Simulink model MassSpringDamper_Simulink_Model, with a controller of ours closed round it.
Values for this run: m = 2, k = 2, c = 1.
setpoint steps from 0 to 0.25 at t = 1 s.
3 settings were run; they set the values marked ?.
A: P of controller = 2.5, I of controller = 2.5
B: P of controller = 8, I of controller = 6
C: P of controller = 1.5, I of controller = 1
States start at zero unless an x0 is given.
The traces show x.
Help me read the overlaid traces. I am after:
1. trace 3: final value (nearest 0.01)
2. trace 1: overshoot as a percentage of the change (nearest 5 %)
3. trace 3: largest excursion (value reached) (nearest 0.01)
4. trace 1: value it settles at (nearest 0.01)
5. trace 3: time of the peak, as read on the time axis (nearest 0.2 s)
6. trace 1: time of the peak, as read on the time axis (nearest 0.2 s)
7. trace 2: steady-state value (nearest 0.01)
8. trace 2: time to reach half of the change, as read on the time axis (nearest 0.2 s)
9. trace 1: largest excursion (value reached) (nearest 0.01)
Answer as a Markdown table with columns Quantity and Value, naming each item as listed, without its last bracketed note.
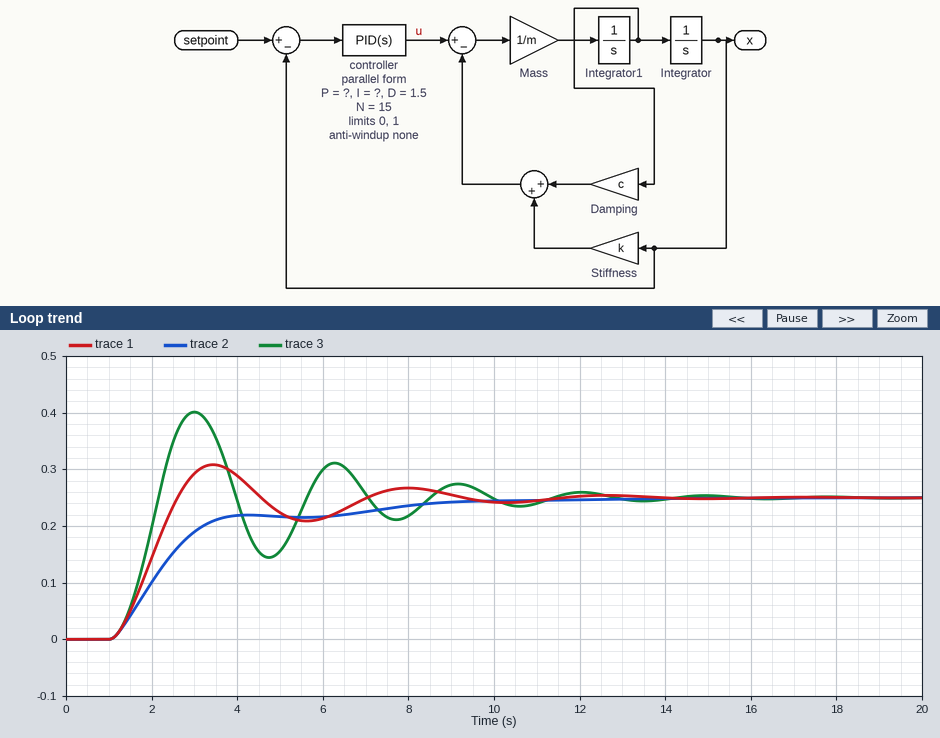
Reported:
| Quantity | Value |
|---|---|
| trace 3: final value | 0.25 |
| trace 1: overshoot as a percentage of the change | 25 % |
| trace 3: largest excursion (value reached) | 0.40 |
| trace 1: value it settles at | 0.25 |
| trace 3: time of the peak, as read on the time axis | 3.0 s |
| trace 1: time of the peak, as read on the time axis | 3.4 s |
| trace 2: steady-state value | 0.25 |
| trace 2: time to reach half of the change, as read on the time axis | 2.2 s |
| trace 1: largest excursion (value reached) | 0.31 |
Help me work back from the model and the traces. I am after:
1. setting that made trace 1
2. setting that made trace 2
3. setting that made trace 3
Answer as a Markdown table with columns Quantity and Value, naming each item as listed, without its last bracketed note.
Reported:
| Quantity | Value |
|---|---|
| setting that made trace 1 | A |
| setting that made trace 2 | C |
| setting that made trace 3 | B |
